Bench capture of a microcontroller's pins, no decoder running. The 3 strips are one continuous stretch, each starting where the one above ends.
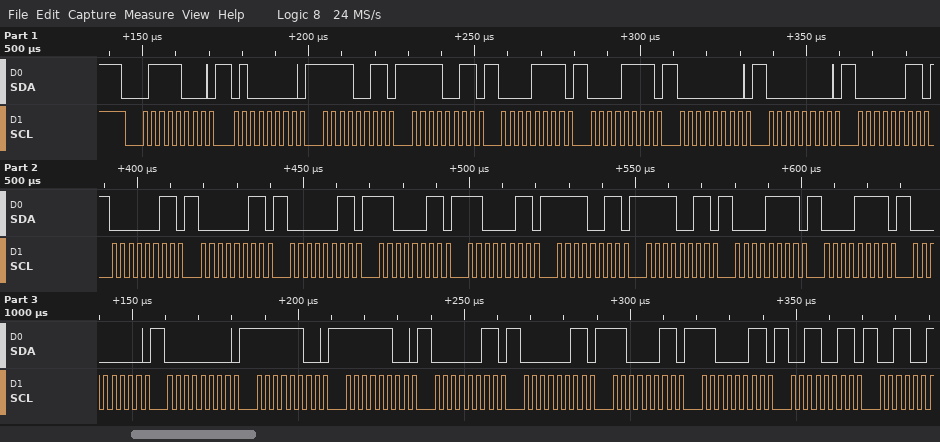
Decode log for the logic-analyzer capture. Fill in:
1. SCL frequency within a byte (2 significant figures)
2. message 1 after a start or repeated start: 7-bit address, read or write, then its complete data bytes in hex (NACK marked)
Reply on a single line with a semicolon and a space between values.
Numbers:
400 kHz; 0x3C write: 40 F3 F3 0F 0F 00 00 03 03 03 03 C3 C3 F3 F3 0F 0F 00 00 FC FC 03 03 C3 C3 33
